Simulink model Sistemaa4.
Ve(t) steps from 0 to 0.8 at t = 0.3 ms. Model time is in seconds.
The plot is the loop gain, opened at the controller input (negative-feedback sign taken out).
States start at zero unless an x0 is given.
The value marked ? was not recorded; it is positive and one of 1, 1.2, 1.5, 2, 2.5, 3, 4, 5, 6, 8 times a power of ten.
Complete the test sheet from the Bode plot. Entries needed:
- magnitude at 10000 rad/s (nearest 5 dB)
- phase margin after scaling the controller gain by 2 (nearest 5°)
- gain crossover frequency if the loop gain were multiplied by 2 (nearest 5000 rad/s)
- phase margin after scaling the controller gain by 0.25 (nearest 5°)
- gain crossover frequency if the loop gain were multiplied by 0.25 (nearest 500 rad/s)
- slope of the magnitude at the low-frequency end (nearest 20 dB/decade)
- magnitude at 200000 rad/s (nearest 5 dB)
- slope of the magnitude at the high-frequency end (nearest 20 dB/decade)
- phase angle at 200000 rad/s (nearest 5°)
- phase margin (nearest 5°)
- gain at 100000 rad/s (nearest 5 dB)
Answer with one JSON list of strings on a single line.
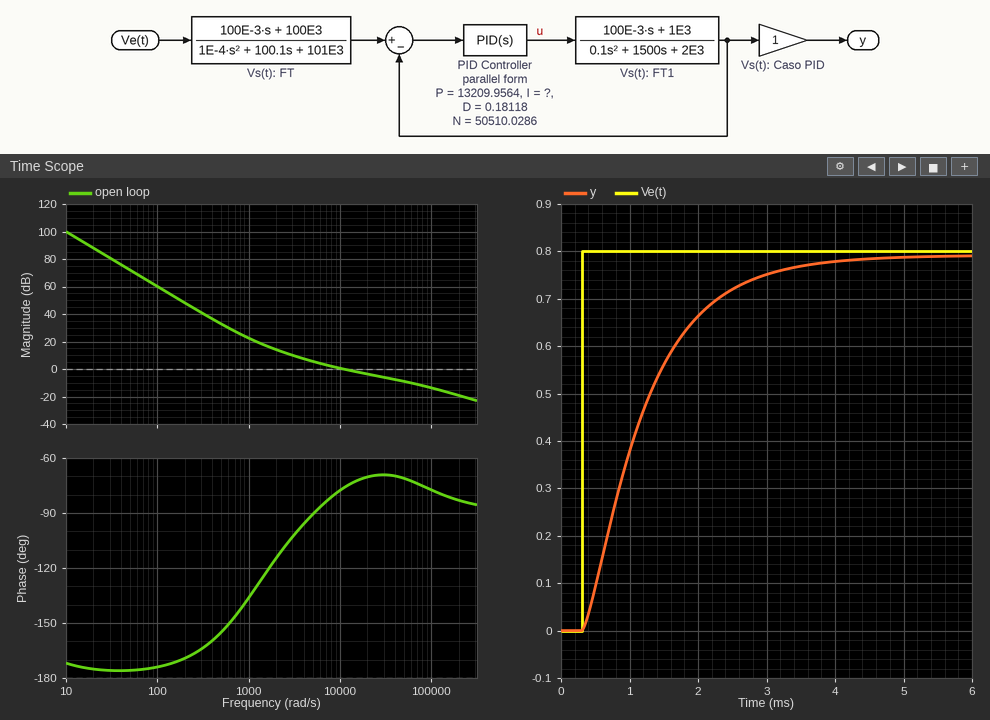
["0 dB", "110°", "30000 rad/s", "70°", "2500 rad/s", "-40 dB/decade", "-20 dB", "-20 dB/decade", "-85°", "105°", "-15 dB"]
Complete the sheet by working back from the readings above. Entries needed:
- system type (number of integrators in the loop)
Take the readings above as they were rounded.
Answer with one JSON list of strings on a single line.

["2"]
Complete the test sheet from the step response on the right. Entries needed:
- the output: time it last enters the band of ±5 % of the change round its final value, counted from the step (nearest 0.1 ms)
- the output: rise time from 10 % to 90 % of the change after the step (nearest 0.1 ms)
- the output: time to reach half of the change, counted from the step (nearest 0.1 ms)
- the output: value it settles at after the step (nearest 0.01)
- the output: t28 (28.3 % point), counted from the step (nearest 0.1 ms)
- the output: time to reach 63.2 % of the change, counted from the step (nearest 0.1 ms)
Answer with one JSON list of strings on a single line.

["2.7 ms", "1.9 ms", "0.7 ms", "0.79", "0.4 ms", "1.0 ms"]
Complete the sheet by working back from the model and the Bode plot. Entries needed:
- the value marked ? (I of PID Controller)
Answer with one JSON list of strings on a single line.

["1.5e+07"]
